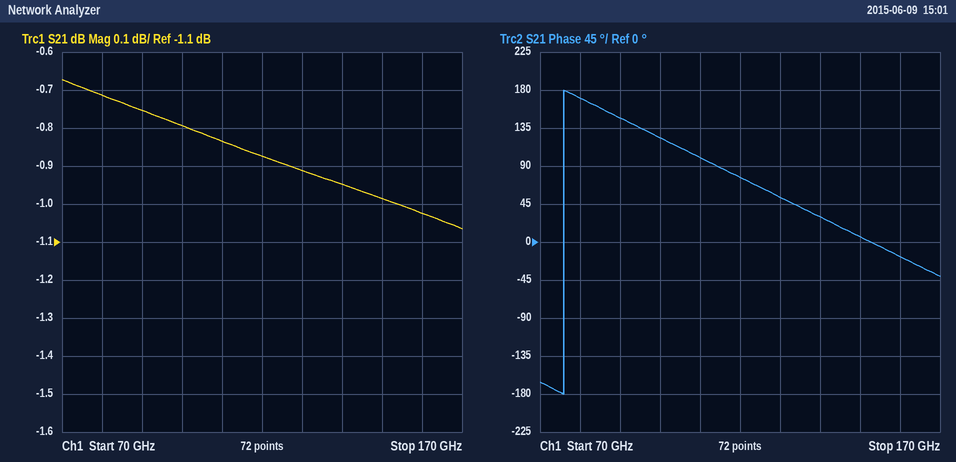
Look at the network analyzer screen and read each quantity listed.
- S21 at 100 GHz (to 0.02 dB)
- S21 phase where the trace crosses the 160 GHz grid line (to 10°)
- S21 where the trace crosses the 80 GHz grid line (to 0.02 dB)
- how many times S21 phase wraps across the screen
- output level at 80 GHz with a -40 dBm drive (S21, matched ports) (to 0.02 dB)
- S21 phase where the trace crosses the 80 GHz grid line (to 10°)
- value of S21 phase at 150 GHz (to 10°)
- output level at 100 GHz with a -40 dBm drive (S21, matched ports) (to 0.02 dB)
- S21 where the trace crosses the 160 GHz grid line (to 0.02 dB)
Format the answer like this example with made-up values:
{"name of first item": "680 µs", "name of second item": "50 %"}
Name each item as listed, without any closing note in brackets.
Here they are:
{"S21 at 100 GHz": "-0.80 dB", "S21 phase where the trace crosses the 160 GHz grid line": "-20°", "S21 where the trace crosses the 80 GHz grid line": "-0.72 dB", "how many times S21 phase wraps across the screen": "1", "output level at 80 GHz with a -40 dBm drive (S21, matched ports)": "-40.72 dBm", "S21 phase where the trace crosses the 80 GHz grid line": "170°", "value of S21 phase at 150 GHz": "10°", "output level at 100 GHz with a -40 dBm drive (S21, matched ports)": "-40.80 dBm", "S21 where the trace crosses the 160 GHz grid line": "-1.02 dB"}
